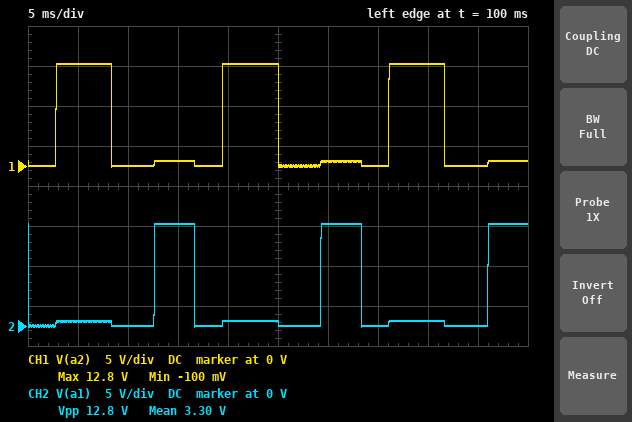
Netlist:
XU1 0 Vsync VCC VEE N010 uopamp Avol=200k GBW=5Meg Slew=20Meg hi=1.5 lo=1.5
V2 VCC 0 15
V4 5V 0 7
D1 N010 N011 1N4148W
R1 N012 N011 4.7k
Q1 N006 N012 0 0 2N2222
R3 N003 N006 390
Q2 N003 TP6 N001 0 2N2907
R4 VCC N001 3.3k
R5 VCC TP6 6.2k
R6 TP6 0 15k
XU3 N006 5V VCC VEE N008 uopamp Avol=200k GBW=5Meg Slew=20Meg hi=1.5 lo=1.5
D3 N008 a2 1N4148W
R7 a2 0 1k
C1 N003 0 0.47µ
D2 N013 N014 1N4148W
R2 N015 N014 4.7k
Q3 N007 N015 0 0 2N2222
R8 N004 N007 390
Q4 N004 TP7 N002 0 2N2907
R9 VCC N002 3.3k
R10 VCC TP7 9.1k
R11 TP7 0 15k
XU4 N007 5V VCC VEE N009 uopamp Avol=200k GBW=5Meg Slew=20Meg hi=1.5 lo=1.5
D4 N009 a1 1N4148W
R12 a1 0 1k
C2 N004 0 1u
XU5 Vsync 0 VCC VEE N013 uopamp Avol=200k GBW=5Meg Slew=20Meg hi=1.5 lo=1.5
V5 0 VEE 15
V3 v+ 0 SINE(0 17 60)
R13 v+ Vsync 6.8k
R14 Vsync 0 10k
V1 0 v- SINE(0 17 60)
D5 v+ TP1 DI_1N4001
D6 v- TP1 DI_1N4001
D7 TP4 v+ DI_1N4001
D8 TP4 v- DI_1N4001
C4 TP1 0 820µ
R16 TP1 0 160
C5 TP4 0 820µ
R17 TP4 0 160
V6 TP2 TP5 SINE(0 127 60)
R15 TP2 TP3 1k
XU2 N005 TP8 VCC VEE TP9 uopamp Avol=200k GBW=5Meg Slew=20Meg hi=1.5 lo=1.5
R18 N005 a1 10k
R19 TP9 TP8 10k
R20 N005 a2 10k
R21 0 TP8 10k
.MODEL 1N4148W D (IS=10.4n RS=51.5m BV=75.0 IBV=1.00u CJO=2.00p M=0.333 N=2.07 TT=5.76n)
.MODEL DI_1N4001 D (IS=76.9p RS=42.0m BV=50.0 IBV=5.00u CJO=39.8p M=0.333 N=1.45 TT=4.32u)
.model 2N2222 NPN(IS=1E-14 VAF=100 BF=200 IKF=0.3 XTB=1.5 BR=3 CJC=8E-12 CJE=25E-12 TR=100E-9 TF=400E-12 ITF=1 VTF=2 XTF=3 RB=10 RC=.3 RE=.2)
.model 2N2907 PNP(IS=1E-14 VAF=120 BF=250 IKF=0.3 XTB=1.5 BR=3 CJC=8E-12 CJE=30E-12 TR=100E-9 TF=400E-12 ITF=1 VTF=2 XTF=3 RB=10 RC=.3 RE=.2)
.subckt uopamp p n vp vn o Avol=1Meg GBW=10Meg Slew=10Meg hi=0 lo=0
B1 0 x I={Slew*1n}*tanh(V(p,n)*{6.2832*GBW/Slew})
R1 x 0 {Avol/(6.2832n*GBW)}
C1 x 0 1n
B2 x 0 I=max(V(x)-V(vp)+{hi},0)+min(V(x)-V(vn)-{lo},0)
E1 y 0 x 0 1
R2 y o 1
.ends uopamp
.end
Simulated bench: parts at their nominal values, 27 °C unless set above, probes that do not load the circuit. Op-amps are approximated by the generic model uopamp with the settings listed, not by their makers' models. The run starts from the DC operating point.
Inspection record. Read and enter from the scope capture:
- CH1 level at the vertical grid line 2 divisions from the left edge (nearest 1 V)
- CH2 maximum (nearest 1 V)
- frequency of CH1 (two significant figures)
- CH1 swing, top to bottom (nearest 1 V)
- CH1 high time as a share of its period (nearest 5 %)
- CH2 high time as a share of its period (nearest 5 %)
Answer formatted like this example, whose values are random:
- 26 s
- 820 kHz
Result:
- 0 V
- 13 V
- 60 Hz
- 13 V
- 35 %
- 25 %
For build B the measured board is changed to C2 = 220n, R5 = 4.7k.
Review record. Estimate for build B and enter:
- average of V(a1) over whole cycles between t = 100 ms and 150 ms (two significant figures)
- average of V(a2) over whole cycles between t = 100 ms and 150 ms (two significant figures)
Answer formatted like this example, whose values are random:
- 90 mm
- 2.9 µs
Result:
- 5.8 V
- 3.9 V
